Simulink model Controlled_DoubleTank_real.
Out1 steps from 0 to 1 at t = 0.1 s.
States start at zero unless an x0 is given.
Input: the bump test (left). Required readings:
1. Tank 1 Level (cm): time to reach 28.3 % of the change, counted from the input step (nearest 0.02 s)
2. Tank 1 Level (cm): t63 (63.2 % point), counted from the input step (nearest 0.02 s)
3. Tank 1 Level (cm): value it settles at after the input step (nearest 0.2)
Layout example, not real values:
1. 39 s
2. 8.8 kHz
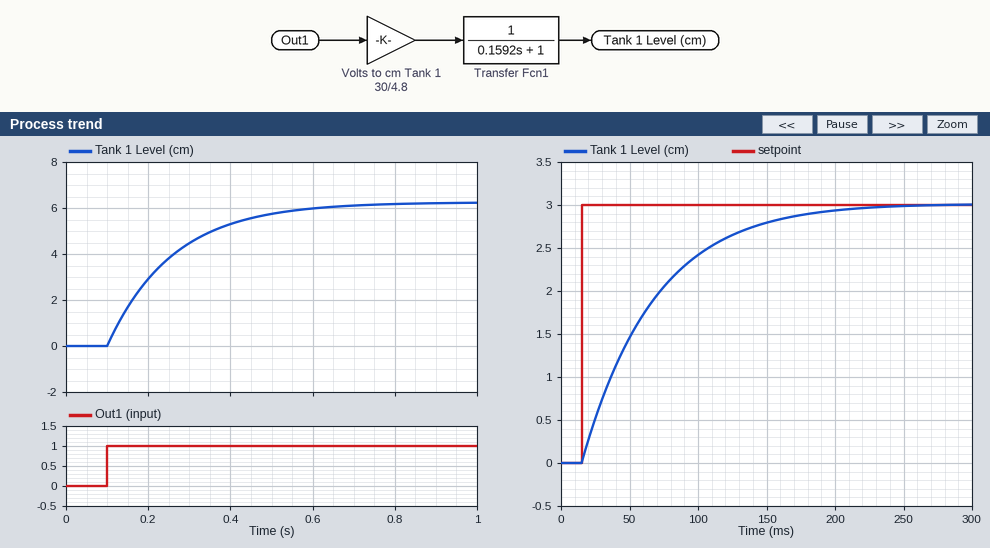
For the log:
1. 0.06 s
2. 0.16 s
3. 6.2
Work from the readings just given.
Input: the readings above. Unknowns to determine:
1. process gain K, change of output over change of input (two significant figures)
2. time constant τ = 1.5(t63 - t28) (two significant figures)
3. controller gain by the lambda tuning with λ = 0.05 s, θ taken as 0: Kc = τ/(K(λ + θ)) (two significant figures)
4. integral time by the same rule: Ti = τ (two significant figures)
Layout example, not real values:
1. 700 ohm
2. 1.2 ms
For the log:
1. 6.2
2. 0.15 s
3. 0.48
4. 0.15 s
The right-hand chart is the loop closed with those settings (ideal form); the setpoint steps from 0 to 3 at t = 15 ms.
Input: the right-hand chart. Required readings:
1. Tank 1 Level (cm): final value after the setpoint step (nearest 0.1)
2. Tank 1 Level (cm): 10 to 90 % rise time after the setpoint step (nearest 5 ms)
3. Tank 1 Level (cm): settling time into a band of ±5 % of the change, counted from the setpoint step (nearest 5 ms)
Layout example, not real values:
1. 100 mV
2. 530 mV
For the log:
1. 3.0
2. 110 ms
3. 150 ms
